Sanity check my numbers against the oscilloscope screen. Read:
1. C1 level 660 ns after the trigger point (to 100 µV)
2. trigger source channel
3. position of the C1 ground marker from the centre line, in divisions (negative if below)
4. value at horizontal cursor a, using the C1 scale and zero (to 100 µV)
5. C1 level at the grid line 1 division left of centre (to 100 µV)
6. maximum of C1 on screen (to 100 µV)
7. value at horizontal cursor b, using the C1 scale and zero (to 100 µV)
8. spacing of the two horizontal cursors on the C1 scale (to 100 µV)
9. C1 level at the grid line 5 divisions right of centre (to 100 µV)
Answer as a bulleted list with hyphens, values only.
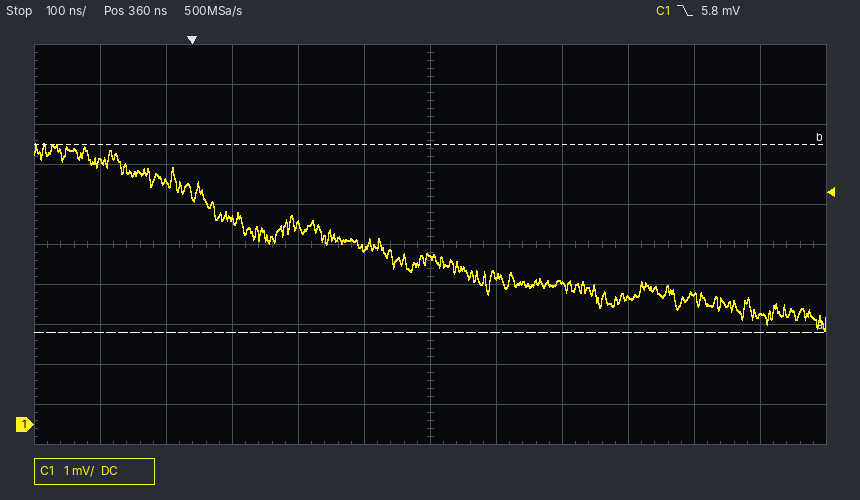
- 3.2 mV
- C1
- -4.5 div
- 2.3 mV
- 4.4 mV
- 7.0 mV
- 7.0 mV
- 4.7 mV
- 2.7 mV
